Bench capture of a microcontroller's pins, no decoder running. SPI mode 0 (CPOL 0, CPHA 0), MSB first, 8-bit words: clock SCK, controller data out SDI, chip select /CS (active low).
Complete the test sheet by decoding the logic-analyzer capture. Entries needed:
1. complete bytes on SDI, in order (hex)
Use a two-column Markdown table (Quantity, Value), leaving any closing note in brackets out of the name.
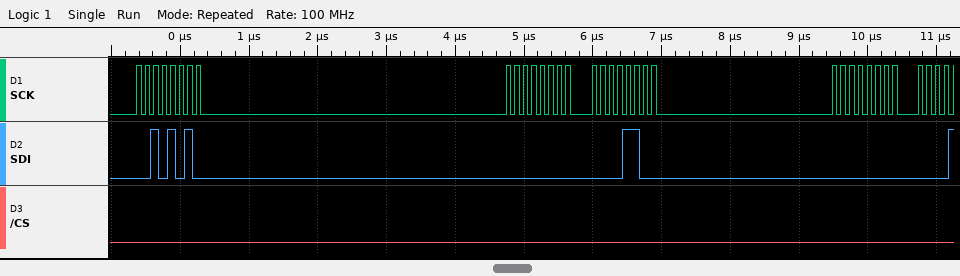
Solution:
| Quantity | Value |
|---|---|
| complete bytes on SDI, in order | 2A 00 0C 00 |
